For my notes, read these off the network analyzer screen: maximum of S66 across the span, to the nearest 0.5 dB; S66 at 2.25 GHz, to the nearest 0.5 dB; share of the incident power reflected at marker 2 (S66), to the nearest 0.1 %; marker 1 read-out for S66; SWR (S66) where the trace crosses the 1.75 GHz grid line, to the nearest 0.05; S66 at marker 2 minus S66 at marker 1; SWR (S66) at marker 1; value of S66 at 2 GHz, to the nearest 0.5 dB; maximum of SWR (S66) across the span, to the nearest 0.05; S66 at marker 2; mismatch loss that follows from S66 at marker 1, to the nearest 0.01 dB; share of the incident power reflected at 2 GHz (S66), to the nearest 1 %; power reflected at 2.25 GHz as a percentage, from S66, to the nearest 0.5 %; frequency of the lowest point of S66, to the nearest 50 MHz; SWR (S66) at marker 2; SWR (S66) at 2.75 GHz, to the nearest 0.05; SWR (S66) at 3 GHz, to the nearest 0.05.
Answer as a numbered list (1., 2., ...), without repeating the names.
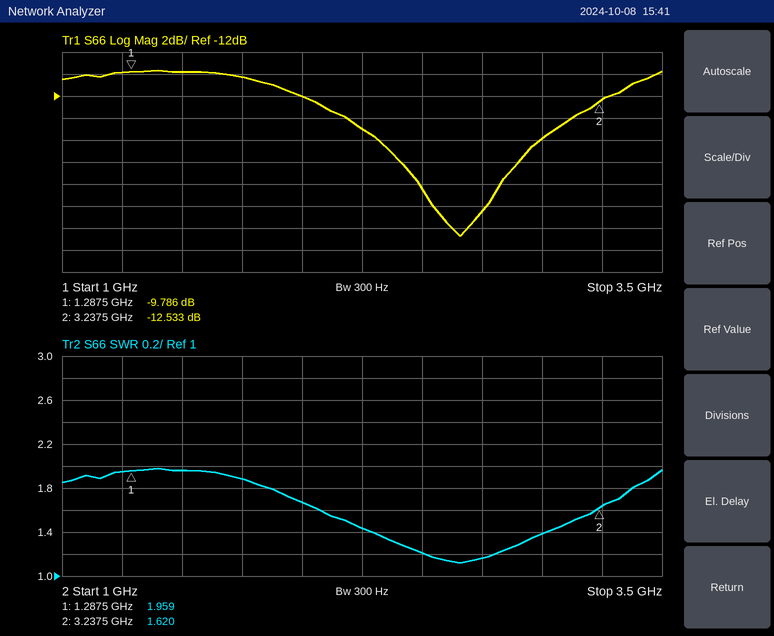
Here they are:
1. -9.5 dB
2. -15.0 dB
3. 5.6 %
4. -9.786 dB
5. 1.90
6. -2.747 dB
7. 1.959
8. -12.0 dB
9. 2.00
10. -12.533 dB
11. 0.48 dB
12. 6 %
13. 3.0 %
14. 2.65 GHz
15. 1.620
16. 1.15
17. 1.40
